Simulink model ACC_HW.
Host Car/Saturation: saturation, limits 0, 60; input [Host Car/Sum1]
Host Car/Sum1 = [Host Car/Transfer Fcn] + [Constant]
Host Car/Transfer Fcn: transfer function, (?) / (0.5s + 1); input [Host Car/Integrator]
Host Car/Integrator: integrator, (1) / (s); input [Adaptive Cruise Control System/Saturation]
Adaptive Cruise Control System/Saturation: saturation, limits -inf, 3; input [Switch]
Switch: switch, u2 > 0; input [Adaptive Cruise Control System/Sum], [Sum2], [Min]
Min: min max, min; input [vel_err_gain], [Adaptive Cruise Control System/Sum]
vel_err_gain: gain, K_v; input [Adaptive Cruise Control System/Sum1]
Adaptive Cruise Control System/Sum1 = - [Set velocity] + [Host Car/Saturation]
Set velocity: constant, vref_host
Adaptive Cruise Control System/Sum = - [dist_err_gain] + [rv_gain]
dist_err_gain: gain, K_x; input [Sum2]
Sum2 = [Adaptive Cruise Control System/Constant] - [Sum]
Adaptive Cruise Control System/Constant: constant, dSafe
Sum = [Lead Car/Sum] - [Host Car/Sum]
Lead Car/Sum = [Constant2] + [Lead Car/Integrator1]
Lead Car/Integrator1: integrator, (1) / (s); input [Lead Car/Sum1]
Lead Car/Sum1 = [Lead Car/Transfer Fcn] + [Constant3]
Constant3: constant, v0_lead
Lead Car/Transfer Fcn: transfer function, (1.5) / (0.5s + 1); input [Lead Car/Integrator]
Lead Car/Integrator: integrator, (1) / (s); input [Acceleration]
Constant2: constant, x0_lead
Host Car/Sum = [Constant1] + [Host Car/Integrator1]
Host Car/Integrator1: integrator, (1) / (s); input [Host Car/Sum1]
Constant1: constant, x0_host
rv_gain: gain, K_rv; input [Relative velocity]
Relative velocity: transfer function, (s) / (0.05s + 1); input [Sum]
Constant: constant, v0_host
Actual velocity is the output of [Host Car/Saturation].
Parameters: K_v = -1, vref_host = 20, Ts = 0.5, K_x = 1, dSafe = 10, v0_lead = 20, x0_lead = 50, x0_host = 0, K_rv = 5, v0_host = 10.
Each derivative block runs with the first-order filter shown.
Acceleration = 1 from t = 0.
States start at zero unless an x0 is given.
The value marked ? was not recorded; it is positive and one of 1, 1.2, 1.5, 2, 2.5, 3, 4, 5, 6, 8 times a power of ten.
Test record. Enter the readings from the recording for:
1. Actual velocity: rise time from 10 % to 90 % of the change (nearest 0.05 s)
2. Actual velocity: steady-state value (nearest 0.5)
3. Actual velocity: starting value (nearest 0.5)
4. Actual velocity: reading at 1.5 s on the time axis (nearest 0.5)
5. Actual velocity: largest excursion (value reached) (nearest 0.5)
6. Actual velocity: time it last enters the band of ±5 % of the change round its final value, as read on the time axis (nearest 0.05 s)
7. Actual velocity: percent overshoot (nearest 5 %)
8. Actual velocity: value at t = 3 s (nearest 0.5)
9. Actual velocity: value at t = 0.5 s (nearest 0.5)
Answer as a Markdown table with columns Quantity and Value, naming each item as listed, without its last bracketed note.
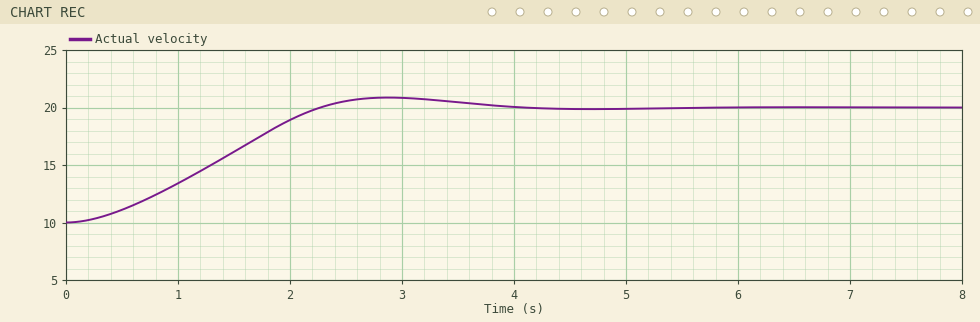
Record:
| Quantity | Value |
|---|---|
| Actual velocity: rise time from 10 % to 90 % of the change | 1.55 s |
| Actual velocity: steady-state value | 20.0 |
| Actual velocity: starting value | 10.0 |
| Actual velocity: reading at 1.5 s on the time axis | 16.0 |
| Actual velocity: largest excursion (value reached) | 21.0 |
| Actual velocity: time it last enters the band of ±5 % of the change round its final value, as read on the time axis | 3.45 s |
| Actual velocity: percent overshoot | 10 % |
| Actual velocity: value at t = 3 s | 21.0 |
| Actual velocity: value at t = 0.5 s | 11.0 |
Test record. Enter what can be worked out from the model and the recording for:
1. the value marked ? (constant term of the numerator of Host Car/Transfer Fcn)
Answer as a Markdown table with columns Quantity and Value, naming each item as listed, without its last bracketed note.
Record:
| Quantity | Value |
|---|---|
| the value marked ? | 2 |
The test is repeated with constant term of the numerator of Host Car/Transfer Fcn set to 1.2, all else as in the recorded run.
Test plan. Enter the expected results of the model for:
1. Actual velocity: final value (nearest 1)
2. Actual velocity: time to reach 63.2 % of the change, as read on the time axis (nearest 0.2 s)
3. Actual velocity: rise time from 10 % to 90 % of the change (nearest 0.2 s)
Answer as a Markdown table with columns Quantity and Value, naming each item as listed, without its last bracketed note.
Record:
| Quantity | Value |
|---|---|
| Actual velocity: final value | 20 |
| Actual velocity: time to reach 63.2 % of the change, as read on the time axis | 2.2 s |
| Actual velocity: rise time from 10 % to 90 % of the change | 2.4 s |
